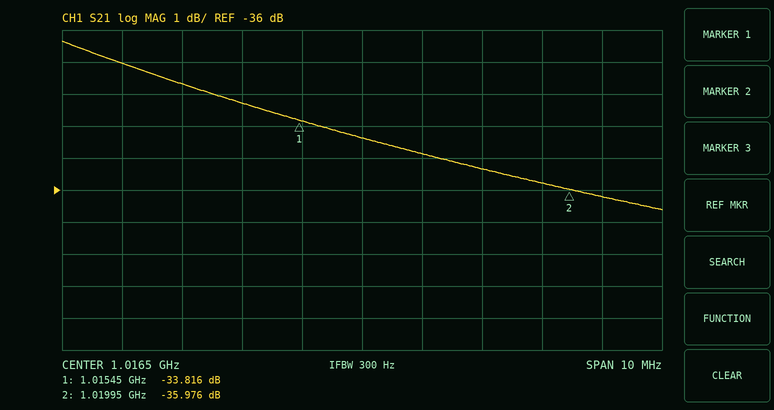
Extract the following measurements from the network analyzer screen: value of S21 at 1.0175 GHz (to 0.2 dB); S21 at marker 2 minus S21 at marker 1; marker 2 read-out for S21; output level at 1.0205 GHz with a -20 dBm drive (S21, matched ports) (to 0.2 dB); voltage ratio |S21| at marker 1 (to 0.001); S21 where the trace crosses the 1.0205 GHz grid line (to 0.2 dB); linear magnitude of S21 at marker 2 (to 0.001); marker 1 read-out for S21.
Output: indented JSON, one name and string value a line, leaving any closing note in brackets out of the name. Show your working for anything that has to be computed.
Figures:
{
  "value of S21 at 1.0175 GHz": "-34.8 dB",
  "S21 at marker 2 minus S21 at marker 1": "-35.976 − (-33.816) = -2.160 dB",
  "marker 2 read-out for S21": "-35.976 dB",
  "output level at 1.0205 GHz with a -20 dBm drive (S21, matched ports)": "-20 dBm + (-36.2 dB) = -56.2 dBm",
  "voltage ratio |S21| at marker 1": "10^(-33.816/20) ≈ 0.020",
  "S21 where the trace crosses the 1.0205 GHz grid line": "-36.2 dB",
  "linear magnitude of S21 at marker 2": "10^(-35.976/20) ≈ 0.016",
  "marker 1 read-out for S21": "-33.816 dB"
}
